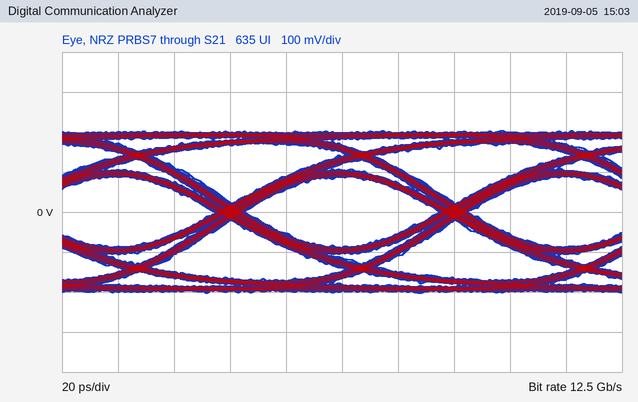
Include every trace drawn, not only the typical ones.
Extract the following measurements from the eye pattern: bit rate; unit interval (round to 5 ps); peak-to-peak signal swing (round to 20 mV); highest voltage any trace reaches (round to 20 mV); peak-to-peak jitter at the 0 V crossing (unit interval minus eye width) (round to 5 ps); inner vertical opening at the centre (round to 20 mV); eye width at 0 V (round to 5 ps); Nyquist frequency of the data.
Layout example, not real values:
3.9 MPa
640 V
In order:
12.5 Gb/s
80 ps
400 mV
200 mV
10 ps
180 mV
70 ps
6.25 GHz
